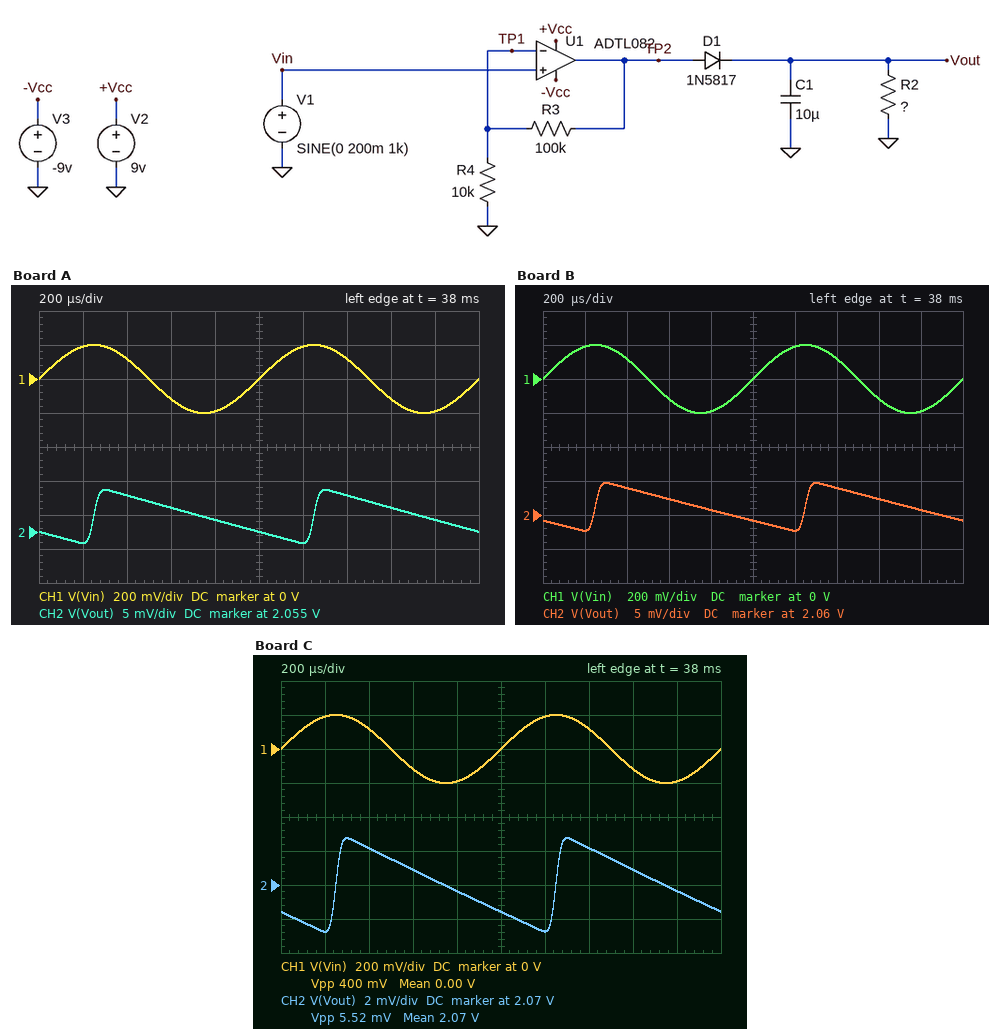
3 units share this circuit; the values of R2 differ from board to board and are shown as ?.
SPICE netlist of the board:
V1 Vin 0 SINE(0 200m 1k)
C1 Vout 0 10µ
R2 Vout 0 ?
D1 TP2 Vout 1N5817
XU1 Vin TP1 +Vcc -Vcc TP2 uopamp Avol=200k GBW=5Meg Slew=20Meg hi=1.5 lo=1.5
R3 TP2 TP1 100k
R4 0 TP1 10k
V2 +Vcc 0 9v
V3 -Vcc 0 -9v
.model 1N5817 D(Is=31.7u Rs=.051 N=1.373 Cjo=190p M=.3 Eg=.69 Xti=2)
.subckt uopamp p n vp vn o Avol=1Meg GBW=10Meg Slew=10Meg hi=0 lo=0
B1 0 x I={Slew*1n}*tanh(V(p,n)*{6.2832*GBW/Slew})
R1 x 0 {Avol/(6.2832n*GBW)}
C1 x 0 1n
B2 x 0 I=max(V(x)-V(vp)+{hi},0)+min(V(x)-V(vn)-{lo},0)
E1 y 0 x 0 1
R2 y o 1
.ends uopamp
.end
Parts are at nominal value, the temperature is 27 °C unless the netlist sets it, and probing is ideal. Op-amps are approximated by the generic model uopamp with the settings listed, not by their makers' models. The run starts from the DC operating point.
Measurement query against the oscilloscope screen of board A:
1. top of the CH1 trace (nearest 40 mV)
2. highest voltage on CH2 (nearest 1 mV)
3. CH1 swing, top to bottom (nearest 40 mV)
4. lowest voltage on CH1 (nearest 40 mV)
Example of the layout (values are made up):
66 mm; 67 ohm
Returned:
200 mV; 2.061 V; 400 mV; -200 mV
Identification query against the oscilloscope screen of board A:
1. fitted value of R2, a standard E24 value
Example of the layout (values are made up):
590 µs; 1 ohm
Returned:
36 kΩ
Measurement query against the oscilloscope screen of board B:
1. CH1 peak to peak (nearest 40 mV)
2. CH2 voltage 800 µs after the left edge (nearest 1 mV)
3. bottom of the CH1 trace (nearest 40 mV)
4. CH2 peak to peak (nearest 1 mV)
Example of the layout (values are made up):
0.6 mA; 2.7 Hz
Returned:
400 mV; 2.061 V; -200 mV; 7 mV
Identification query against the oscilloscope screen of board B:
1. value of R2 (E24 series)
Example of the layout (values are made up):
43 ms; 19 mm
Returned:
43 kΩ
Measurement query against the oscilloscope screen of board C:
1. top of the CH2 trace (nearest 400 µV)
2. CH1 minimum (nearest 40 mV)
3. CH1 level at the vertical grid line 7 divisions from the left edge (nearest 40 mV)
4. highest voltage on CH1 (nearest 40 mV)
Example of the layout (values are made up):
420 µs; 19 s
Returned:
2.0728 V; -200 mV; 120 mV; 200 mV
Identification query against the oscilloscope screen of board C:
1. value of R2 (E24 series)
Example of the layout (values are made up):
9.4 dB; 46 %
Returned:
68 kΩ
